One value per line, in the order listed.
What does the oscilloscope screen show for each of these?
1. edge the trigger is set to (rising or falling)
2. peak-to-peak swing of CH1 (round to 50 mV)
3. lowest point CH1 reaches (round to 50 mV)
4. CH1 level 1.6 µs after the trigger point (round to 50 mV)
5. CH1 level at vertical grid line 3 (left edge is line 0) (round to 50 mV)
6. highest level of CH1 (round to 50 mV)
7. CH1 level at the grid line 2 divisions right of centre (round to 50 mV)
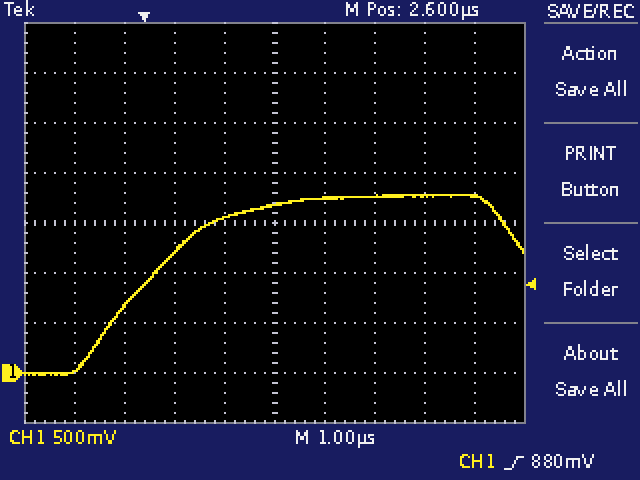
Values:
rising
1.80 V
0 mV
1.55 V
1.20 V
1.80 V
1.75 V
